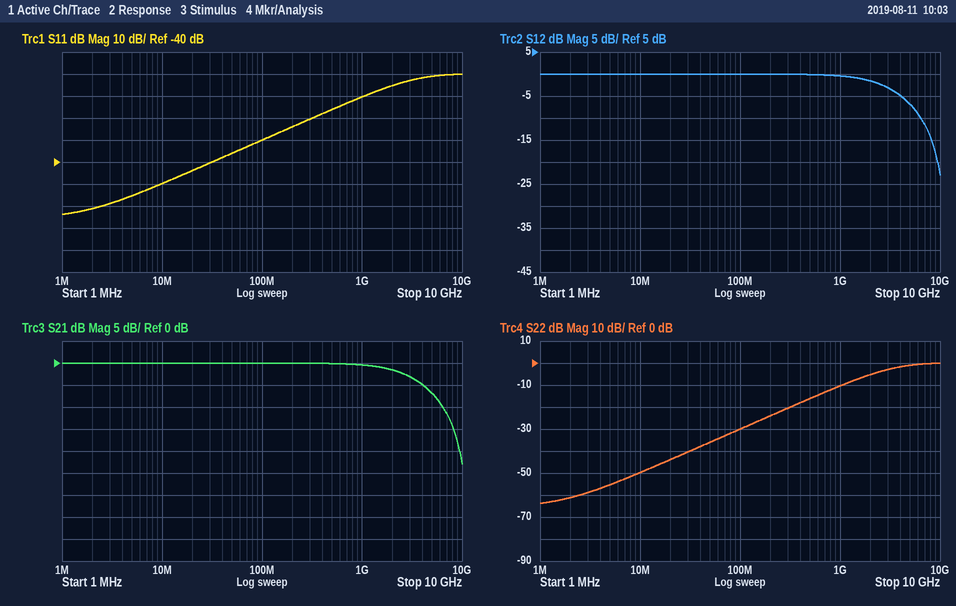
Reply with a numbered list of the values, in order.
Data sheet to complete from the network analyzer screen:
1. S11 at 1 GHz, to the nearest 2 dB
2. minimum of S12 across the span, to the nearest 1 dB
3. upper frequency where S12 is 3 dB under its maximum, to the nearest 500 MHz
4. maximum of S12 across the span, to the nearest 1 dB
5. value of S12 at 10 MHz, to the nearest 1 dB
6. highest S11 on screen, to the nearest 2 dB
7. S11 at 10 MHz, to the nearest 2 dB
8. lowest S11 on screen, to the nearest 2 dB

1. -10 dB
2. -23 dB
3. 3.0 GHz
4. 0 dB
5. 0 dB
6. 0 dB
7. -50 dB
8. -64 dB
